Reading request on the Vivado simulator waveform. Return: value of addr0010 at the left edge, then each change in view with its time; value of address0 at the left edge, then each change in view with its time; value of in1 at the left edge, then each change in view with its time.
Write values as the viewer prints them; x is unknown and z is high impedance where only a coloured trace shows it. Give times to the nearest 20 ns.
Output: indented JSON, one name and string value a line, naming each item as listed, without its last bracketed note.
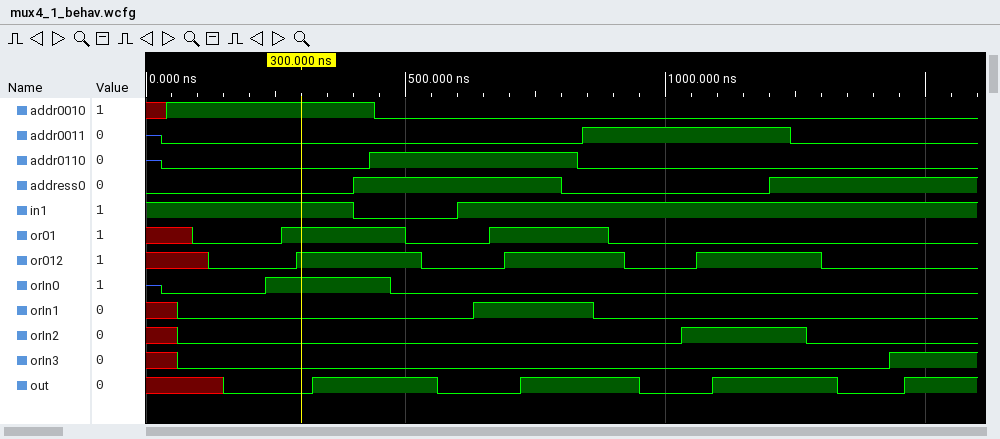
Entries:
{
  "value of addr0010 at the left edge, then each change in view with its time": "x, 1 at 40 ns, 0 at 440 ns",
  "value of address0 at the left edge, then each change in view with its time": "0, 1 at 400 ns, 0 at 800 ns, 1 at 1200 ns",
  "value of in1 at the left edge, then each change in view with its time": "1, 0 at 400 ns, 1 at 600 ns"
}
